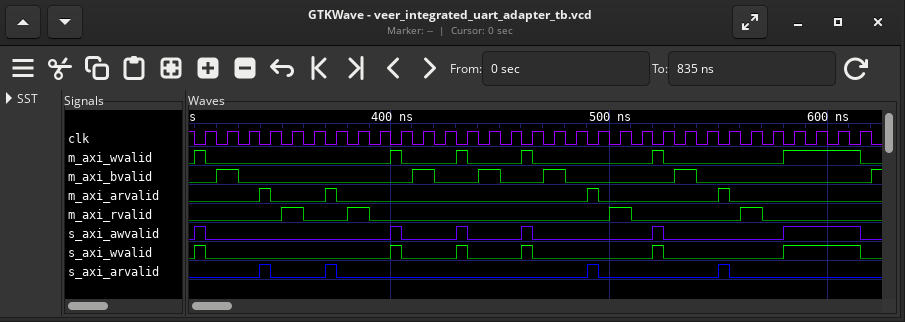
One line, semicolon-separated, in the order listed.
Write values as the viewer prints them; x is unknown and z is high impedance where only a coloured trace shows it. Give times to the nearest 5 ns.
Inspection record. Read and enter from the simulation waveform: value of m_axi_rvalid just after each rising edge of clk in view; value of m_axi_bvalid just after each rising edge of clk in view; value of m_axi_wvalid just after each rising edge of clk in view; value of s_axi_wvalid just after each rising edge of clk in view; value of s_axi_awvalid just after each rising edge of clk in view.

0 0 0 0 1 0 0 1 0 0 0 0 0 0 0 0 0 0 0 1 0 0 0 0 0 1 0 0 0 0 0; 0 1 0 0 0 0 0 0 0 0 1 0 0 1 0 0 1 0 0 0 0 0 1 0 0 0 0 0 0 0 0; 0 0 0 0 0 0 0 0 0 0 0 0 0 0 0 0 0 0 0 0 0 0 0 0 0 0 0 1 1 1 0; 0 0 0 0 0 0 0 0 0 0 0 0 0 0 0 0 0 0 0 0 0 0 0 0 0 0 0 1 1 1 0; 0 0 0 0 0 0 0 0 0 0 0 0 0 0 0 0 0 0 0 0 0 0 0 0 0 0 0 1 1 1 0
